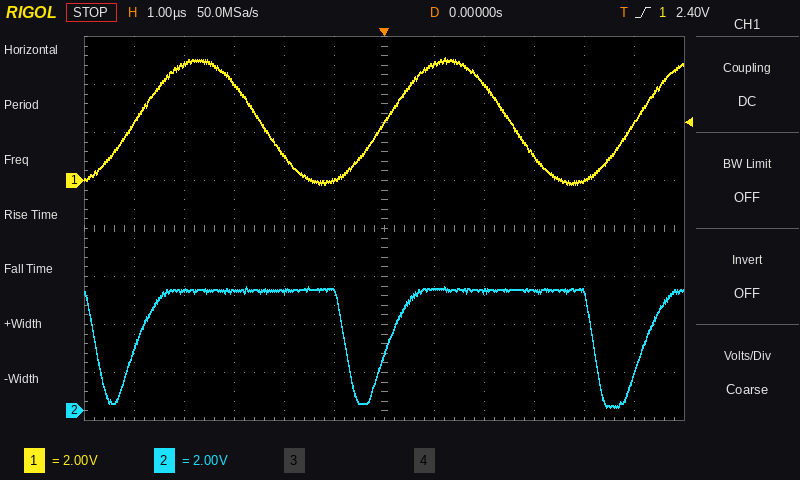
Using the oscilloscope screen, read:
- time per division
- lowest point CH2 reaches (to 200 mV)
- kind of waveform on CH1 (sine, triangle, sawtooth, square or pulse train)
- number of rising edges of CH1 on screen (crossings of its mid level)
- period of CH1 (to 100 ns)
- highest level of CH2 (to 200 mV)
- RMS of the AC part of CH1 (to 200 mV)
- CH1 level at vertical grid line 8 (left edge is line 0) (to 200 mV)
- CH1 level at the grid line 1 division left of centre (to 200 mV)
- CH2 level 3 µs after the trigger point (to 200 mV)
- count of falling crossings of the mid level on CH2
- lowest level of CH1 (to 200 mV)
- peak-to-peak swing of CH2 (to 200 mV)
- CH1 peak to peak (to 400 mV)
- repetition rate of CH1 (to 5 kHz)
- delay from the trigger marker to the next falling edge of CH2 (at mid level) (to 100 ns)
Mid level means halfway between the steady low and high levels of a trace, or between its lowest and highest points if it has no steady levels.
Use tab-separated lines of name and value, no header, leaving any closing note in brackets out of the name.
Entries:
time per division	1 µs
lowest point CH2 reaches	200 mV
kind of waveform on CH1	sine
number of rising edges of CH1 on screen	3
period of CH1	5.0 µs
highest level of CH2	5.2 V
RMS of the AC part of CH1	1.8 V
CH1 level at vertical grid line 8 (left edge is line 0)	4.0 V
CH1 level at the grid line 1 division left of centre	0.0 V
CH2 level 3 µs after the trigger point	5.0 V
count of falling crossings of the mid level on CH2	3
lowest level of CH1	-200 mV
peak-to-peak swing of CH2	5.0 V
CH1 peak to peak	5.2 V
repetition rate of CH1	200 kHz
delay from the trigger marker to the next falling edge of CH2 (at mid level)	4.2 µs
